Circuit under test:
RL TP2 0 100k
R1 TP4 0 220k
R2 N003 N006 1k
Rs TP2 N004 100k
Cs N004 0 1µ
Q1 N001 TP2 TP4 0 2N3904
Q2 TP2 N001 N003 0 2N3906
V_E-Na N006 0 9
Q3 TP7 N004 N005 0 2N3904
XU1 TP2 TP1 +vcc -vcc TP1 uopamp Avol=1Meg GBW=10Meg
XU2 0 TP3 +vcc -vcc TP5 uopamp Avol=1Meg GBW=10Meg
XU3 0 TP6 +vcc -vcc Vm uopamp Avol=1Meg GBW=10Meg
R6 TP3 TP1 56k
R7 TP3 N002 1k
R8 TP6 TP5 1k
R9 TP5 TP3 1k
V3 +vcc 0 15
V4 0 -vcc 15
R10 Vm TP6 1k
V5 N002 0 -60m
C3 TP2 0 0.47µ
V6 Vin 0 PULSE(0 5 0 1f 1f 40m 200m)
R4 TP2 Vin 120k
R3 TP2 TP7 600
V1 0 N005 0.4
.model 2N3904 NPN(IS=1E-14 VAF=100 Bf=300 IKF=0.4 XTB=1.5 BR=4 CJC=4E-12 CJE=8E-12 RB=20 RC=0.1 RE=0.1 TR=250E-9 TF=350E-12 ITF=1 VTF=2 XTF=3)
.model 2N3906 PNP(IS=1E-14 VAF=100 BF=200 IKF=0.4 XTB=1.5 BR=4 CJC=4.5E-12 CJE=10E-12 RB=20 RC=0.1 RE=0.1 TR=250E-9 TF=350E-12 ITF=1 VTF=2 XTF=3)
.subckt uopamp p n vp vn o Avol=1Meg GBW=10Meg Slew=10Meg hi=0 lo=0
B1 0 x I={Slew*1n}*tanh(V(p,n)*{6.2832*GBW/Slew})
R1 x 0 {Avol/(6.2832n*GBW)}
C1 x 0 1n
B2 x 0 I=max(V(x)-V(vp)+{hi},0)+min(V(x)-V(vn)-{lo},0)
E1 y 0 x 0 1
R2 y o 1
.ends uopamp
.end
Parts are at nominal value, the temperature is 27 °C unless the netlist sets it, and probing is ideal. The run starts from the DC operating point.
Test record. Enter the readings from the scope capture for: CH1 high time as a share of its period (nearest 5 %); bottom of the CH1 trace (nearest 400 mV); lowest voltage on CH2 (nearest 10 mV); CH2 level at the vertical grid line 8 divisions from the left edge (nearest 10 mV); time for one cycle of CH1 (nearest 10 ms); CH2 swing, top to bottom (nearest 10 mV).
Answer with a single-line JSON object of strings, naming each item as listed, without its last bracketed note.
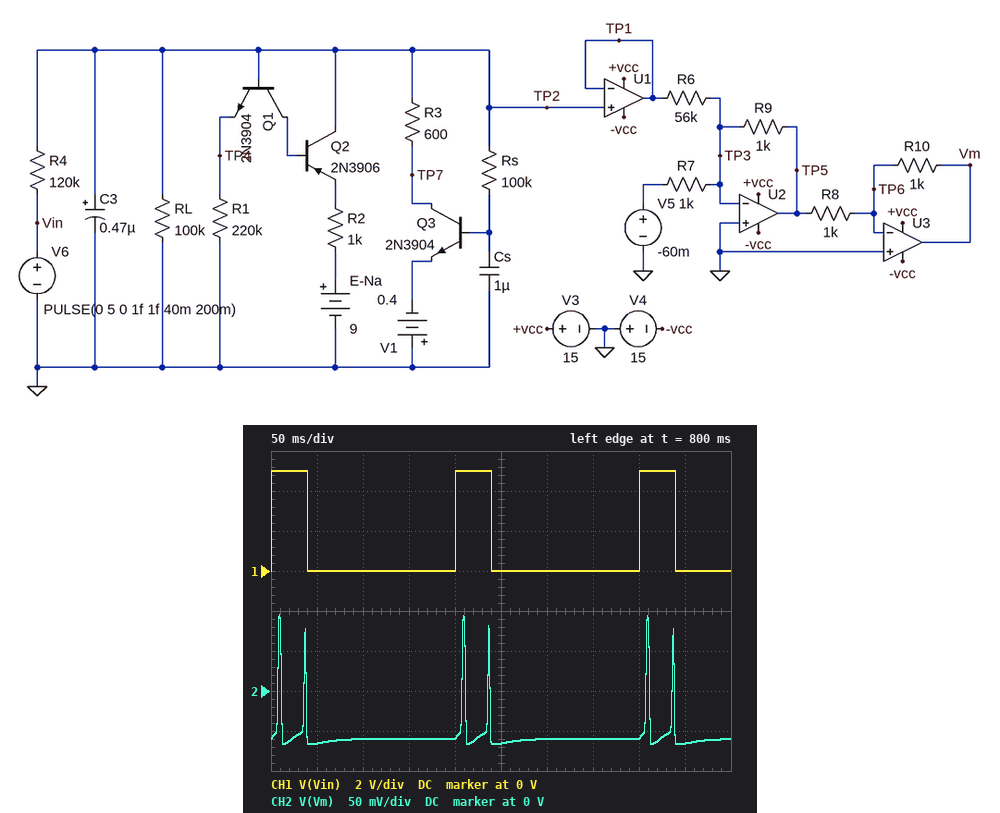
{"CH1 high time as a share of its period": "20 %", "bottom of the CH1 trace": "0 V", "lowest voltage on CH2": "-70 mV", "CH2 level at the vertical grid line 8 divisions from the left edge": "-60 mV", "time for one cycle of CH1": "200 ms", "CH2 swing, top to bottom": "160 mV"}
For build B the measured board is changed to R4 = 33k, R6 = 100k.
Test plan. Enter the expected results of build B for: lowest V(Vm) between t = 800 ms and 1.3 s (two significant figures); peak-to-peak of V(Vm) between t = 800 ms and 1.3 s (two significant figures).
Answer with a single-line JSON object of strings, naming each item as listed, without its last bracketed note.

{"lowest V(Vm) between t = 800 ms and 1.3 s": "-64 mV", "peak-to-peak of V(Vm) between t = 800 ms and 1.3 s": "89 mV"}
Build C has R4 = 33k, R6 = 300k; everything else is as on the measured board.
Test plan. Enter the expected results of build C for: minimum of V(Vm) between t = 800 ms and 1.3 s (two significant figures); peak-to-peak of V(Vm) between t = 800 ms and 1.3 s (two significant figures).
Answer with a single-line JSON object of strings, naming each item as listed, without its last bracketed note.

{"minimum of V(Vm) between t = 800 ms and 1.3 s": "-61 mV", "peak-to-peak of V(Vm) between t = 800 ms and 1.3 s": "30 mV"}
